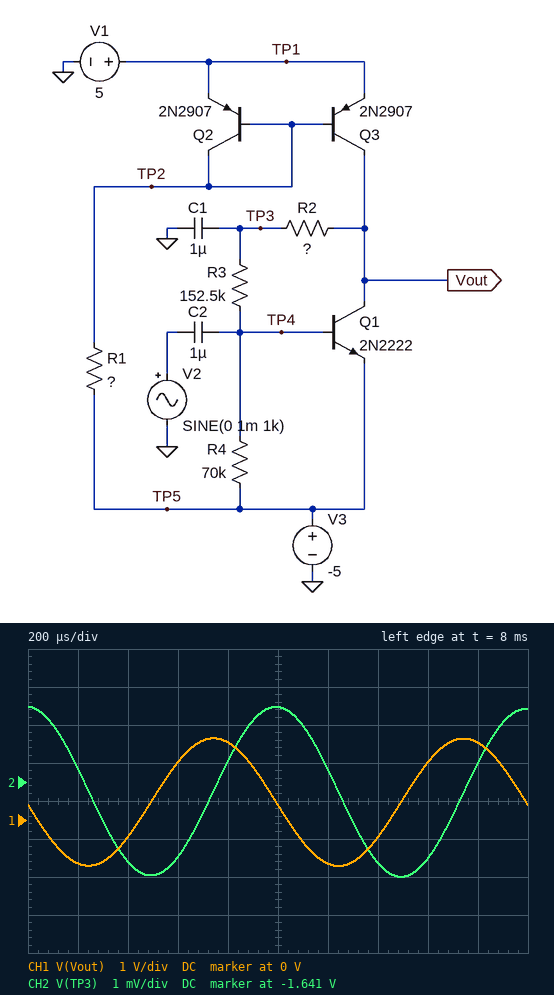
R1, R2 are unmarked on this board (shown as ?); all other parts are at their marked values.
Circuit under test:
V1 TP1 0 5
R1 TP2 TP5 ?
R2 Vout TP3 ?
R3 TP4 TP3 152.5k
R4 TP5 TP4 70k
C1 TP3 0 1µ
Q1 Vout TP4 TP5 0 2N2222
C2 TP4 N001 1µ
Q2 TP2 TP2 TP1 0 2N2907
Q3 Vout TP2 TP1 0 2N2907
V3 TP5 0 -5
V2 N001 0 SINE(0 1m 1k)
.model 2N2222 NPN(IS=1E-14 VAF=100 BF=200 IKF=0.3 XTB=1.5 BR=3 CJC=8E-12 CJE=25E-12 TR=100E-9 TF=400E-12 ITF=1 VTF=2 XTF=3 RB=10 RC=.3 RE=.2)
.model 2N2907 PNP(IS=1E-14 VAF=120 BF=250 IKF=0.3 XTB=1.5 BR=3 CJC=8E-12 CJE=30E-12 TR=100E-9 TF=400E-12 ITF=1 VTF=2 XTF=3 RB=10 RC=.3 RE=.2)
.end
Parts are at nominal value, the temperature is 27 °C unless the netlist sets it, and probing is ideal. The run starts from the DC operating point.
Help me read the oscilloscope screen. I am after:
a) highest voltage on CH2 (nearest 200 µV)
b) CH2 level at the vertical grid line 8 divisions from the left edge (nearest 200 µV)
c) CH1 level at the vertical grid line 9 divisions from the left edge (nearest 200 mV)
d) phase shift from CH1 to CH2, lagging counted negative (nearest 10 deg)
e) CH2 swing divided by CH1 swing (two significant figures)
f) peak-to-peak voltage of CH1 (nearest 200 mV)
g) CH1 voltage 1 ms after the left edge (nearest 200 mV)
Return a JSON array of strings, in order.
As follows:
["-1.6390 V", "-1.6430 V", "2.0 V", "-90 deg", "0.0013", "3.4 V", "400 mV"]
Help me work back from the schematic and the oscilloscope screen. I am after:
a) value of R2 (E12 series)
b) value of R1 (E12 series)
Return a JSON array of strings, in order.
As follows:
["120 kΩ", "5.6 kΩ"]
